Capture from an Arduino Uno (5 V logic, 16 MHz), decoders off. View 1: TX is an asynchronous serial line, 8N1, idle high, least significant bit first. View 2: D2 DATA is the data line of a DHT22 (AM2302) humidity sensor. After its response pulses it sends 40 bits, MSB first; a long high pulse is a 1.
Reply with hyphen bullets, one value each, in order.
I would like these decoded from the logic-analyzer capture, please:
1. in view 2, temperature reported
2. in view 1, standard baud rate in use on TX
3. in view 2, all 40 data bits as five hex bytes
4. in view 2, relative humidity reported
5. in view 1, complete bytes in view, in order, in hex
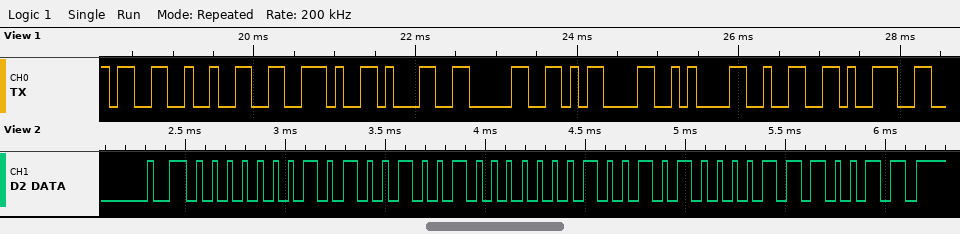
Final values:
- 29.6 °C
- 9600 baud
- 01 49 01 28 73
- 32.9 %
- 33 32 2E 31 30 0D 0A 32 39
